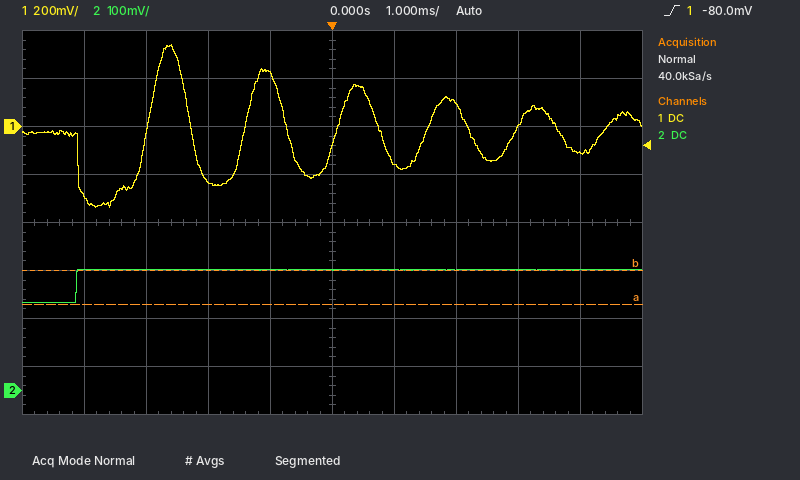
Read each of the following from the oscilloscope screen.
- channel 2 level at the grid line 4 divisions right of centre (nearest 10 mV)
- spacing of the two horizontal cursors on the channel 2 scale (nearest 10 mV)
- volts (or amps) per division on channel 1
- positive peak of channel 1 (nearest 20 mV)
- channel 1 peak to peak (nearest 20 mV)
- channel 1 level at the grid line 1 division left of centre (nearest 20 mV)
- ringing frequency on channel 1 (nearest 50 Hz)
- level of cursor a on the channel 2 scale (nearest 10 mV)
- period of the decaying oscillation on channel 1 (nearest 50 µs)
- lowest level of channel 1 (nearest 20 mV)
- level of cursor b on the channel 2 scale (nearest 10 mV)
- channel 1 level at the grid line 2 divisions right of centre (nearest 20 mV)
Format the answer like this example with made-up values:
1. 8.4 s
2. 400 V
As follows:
1. 250 mV
2. 70 mV
3. 200 mV
4. 340 mV
5. 680 mV
6. 220 mV
7. 700 Hz
8. 180 mV
9. 1.45 ms
10. -340 mV
11. 250 mV
12. 100 mV
